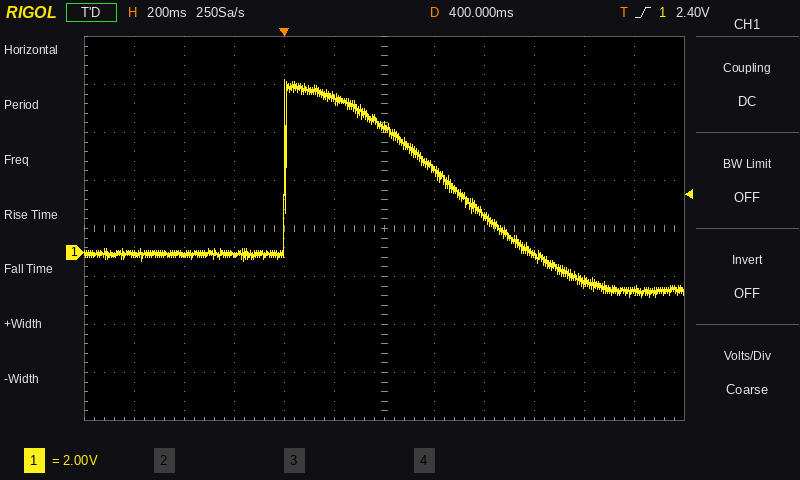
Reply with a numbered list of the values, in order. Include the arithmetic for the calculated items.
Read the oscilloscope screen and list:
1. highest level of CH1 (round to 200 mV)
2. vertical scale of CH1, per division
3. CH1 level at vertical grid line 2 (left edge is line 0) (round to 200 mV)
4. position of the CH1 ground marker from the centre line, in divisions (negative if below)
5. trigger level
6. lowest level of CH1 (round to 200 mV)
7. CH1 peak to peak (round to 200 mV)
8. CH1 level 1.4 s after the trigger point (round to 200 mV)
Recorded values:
1. 7.2 V
2. 2 V
3. 0.0 V
4. -0.5 div
5. 2.40 V
6. -1.8 V
7. 7.2 V − (-1.8 V) = 9.0 V
8. -1.6 V
